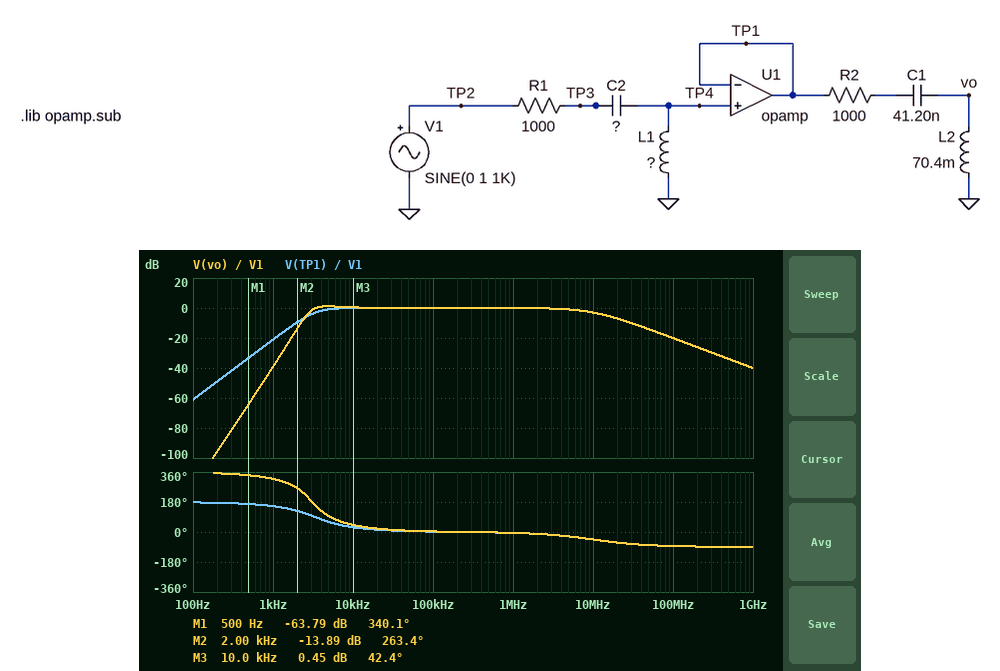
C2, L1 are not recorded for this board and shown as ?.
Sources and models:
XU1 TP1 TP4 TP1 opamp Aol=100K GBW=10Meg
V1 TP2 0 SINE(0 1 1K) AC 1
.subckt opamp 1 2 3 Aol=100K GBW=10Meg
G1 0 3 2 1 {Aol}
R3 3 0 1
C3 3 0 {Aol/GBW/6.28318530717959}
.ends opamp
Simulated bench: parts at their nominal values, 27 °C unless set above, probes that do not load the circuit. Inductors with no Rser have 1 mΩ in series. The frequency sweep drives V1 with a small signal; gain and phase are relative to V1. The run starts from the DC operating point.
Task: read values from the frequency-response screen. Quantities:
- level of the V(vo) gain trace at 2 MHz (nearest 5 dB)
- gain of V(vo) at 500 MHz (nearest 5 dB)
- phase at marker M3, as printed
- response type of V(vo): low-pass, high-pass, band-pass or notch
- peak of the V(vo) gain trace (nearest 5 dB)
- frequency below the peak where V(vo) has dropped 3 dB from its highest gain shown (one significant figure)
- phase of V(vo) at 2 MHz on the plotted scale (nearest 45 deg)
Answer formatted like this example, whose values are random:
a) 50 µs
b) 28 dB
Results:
a) 0 dB
b) -35 dB
c) 42.4 deg
d) band-pass
e) 0 dB
f) 3 kHz
g) 0 deg
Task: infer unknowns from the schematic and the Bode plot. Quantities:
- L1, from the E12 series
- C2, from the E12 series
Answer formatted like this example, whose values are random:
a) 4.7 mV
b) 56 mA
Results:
a) 33 mH
b) 68 nF
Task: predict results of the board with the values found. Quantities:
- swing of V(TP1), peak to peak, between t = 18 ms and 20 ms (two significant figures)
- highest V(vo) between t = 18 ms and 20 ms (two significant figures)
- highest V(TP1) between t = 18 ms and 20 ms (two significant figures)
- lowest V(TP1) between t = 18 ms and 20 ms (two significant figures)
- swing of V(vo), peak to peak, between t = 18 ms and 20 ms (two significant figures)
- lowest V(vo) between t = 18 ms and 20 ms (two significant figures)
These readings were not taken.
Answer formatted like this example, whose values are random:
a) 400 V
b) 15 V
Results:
a) 180 mV
b) 11 mV
c) 88 mV
d) -88 mV
e) 22 mV
f) -11 mV
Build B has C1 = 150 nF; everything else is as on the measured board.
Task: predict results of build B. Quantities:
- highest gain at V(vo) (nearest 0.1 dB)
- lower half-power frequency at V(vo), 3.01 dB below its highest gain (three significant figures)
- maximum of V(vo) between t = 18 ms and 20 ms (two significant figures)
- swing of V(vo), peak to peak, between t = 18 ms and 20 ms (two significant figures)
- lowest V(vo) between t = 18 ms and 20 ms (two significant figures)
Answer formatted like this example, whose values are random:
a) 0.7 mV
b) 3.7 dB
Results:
a) 0 dB
b) 3.52 kHz
c) 33 mV
d) 66 mV
e) -33 mV
